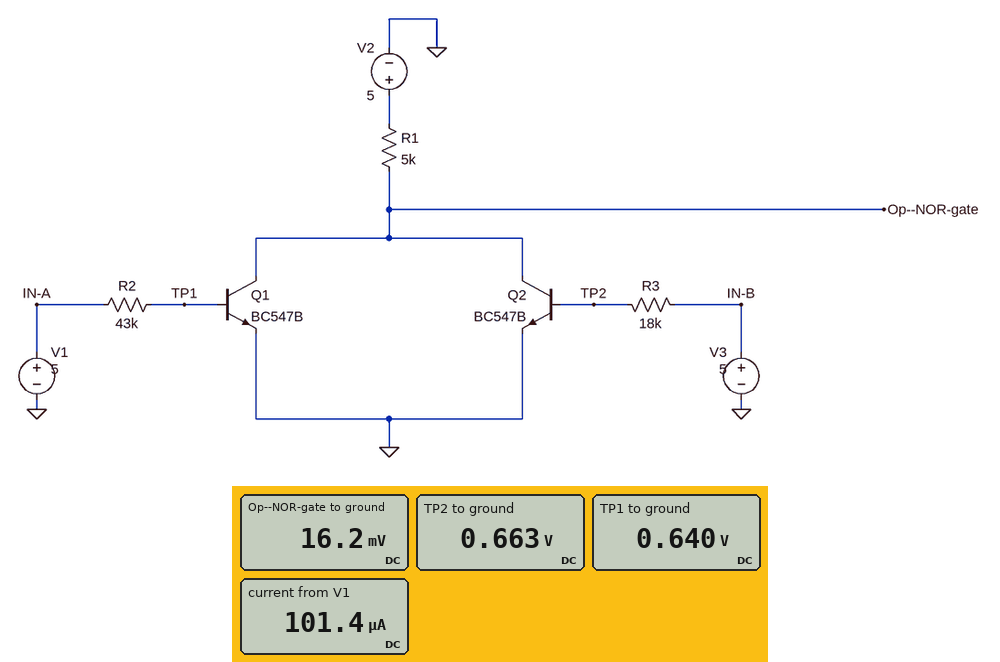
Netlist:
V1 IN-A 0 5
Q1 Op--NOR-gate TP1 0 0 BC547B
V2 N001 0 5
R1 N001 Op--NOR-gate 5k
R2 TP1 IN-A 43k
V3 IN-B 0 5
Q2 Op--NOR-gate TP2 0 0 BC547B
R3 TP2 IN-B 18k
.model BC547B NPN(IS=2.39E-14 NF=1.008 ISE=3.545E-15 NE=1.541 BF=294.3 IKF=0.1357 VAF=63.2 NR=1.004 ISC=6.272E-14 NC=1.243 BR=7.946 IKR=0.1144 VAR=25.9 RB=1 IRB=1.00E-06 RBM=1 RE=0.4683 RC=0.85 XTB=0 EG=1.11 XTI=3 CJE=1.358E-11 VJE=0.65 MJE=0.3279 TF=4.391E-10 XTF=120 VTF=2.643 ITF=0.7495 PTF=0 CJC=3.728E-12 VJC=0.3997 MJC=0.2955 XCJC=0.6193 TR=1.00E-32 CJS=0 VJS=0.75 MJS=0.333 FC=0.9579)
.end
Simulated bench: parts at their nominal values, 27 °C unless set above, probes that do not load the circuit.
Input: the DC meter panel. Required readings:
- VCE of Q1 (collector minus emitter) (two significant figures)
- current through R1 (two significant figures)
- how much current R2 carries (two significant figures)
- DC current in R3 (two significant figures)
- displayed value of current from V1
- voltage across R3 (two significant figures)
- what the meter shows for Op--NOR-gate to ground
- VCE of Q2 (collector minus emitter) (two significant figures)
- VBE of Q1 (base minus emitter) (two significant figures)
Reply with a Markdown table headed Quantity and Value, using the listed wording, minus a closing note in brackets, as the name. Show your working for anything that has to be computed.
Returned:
| Quantity | Value |
|---|---|
| VCE of Q1 (collector minus emitter) | 16.2 mV = 16 mV |
| current through R1 | (5 V - 16.2 mV) / 5 kΩ = 1.0 mA |
| how much current R2 carries | (5 V - 640 mV) / 43 kΩ = 100 µA |
| DC current in R3 | (5 V - 663 mV) / 18 kΩ = 240 µA |
| displayed value of current from V1 | 101.4 µA |
| voltage across R3 | 5 V - 663 mV = 4.3 V |
| what the meter shows for Op--NOR-gate to ground | 16.2 mV |
| VCE of Q2 (collector minus emitter) | 16.2 mV = 16 mV |
| VBE of Q1 (base minus emitter) | 640 mV = 640 mV |
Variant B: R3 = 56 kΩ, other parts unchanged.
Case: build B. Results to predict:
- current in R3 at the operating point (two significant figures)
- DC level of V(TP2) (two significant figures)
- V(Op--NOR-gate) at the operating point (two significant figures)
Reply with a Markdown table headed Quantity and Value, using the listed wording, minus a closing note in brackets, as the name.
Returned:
| Quantity | Value |
|---|---|
| current in R3 at the operating point | 78 µA |
| DC level of V(TP2) | 640 mV |
| V(Op--NOR-gate) at the operating point | 22 mV |
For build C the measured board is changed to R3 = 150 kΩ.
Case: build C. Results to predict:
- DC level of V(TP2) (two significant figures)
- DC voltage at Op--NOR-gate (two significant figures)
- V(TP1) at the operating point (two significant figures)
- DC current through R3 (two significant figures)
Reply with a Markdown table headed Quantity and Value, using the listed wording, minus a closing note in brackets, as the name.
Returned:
| Quantity | Value |
|---|---|
| DC level of V(TP2) | 620 mV |
| DC voltage at Op--NOR-gate | 27 mV |
| V(TP1) at the operating point | 650 mV |
| DC current through R3 | 29 µA |
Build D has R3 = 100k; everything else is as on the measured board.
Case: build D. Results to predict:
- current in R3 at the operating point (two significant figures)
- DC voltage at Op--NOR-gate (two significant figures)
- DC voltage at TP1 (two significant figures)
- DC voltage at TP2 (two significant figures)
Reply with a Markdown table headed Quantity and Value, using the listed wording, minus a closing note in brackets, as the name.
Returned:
| Quantity | Value |
|---|---|
| current in R3 at the operating point | 44 µA |
| DC voltage at Op--NOR-gate | 25 mV |
| DC voltage at TP1 | 650 mV |
| DC voltage at TP2 | 630 mV |
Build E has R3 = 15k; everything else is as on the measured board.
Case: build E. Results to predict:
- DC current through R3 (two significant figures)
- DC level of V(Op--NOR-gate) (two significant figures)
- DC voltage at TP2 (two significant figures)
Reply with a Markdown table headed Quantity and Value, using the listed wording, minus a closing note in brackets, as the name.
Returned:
| Quantity | Value |
|---|---|
| DC current through R3 | 290 µA |
| DC level of V(Op--NOR-gate) | 15 mV |
| DC voltage at TP2 | 670 mV |
